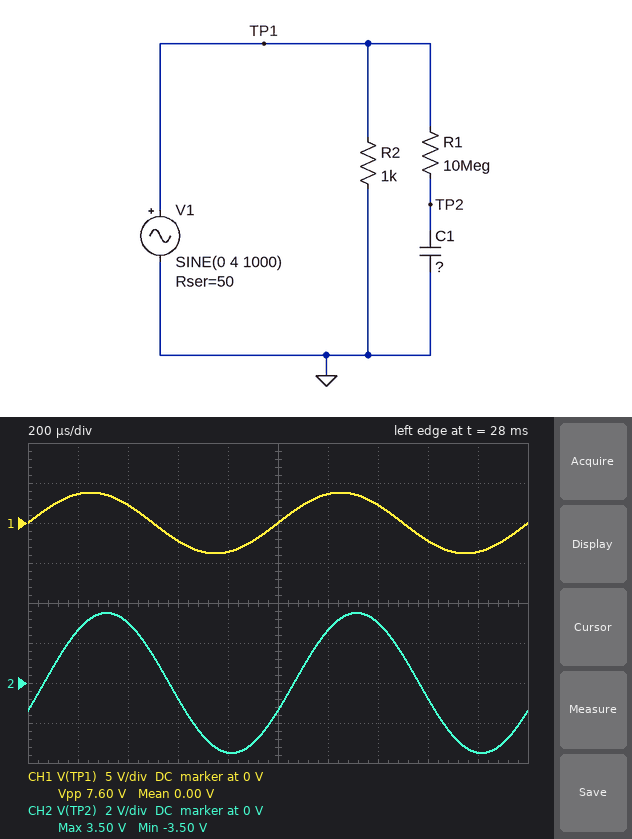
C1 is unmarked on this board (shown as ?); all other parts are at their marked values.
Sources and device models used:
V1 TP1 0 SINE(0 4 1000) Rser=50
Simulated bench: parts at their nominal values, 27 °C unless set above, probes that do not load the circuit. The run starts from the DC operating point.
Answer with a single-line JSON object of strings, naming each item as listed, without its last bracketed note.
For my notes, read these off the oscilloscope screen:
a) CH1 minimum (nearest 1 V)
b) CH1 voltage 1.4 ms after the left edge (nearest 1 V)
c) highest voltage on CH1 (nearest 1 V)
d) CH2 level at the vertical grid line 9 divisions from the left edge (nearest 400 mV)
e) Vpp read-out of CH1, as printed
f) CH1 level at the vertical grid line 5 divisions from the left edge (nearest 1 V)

{"CH1 minimum": "-4 V", "CH1 voltage 1.4 ms after the left edge": "2 V", "highest voltage on CH1": "4 V", "CH2 level at the vertical grid line 9 divisions from the left edge": "-3.6 V", "Vpp read-out of CH1, as printed": "7.60 V", "CH1 level at the vertical grid line 5 divisions from the left edge": "0 V"}
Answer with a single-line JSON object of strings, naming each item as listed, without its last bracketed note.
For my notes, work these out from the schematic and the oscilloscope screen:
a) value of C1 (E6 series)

{"value of C1": "6.8 pF"}
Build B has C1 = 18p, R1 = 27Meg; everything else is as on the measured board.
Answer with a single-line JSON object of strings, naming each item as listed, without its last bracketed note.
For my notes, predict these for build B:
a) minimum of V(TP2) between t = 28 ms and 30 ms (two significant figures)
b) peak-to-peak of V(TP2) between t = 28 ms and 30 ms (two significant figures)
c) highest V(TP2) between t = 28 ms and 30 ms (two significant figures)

{"minimum of V(TP2) between t = 28 ms and 30 ms": "-1.2 V", "peak-to-peak of V(TP2) between t = 28 ms and 30 ms": "2.4 V", "highest V(TP2) between t = 28 ms and 30 ms": "1.2 V"}
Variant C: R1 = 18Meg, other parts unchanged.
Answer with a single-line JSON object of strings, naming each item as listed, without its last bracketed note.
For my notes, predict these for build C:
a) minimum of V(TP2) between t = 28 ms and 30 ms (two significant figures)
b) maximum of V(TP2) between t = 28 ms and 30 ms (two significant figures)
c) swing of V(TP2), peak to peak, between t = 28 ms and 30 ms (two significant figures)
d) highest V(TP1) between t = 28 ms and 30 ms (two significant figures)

{"minimum of V(TP2) between t = 28 ms and 30 ms": "-3.0 V", "maximum of V(TP2) between t = 28 ms and 30 ms": "3.0 V", "swing of V(TP2), peak to peak, between t = 28 ms and 30 ms": "6.0 V", "highest V(TP1) between t = 28 ms and 30 ms": "3.8 V"}
